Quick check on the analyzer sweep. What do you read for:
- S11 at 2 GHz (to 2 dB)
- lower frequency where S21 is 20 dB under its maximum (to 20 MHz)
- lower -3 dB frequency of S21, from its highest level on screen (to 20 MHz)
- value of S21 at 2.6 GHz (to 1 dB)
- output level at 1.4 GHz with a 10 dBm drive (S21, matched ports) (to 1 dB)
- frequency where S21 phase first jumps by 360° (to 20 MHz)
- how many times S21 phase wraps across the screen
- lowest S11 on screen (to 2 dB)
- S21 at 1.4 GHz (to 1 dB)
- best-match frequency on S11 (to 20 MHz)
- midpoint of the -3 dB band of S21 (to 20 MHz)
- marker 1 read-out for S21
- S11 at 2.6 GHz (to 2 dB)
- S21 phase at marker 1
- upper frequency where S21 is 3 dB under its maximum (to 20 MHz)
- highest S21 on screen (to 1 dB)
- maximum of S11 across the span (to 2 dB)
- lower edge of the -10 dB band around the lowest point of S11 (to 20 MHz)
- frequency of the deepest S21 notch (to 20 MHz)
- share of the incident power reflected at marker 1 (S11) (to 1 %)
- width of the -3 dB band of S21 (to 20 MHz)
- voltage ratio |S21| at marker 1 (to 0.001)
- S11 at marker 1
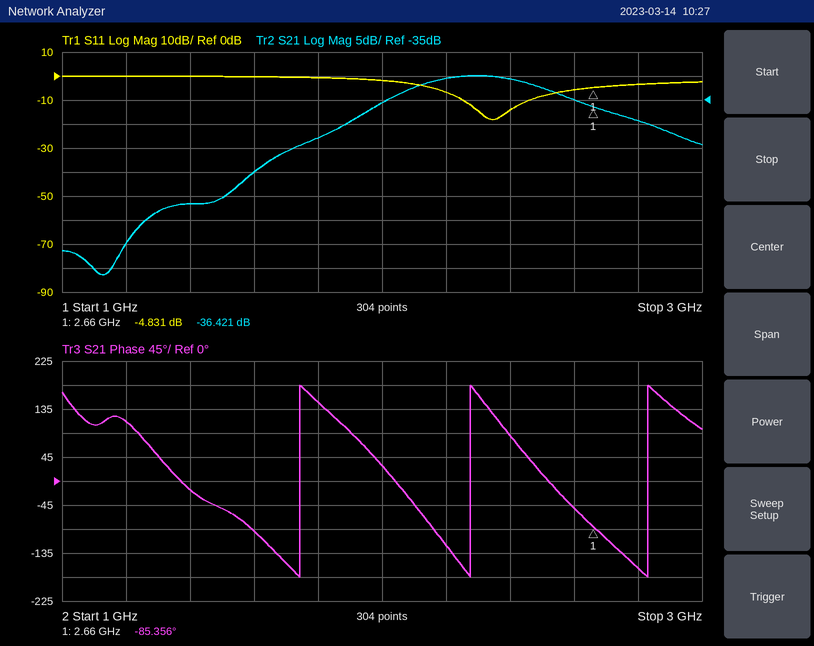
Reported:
-2 dB
1.60 GHz
2.08 GHz
-35 dB
-47 dBm
1.74 GHz
3
-18 dB
-57 dB
2.34 GHz
2.30 GHz
-36.421 dB
-6 dB
-85.356°
2.52 GHz
-30 dB
0 dB
2.26 GHz
1.12 GHz
33 %
440 MHz
0.015
-4.831 dB
